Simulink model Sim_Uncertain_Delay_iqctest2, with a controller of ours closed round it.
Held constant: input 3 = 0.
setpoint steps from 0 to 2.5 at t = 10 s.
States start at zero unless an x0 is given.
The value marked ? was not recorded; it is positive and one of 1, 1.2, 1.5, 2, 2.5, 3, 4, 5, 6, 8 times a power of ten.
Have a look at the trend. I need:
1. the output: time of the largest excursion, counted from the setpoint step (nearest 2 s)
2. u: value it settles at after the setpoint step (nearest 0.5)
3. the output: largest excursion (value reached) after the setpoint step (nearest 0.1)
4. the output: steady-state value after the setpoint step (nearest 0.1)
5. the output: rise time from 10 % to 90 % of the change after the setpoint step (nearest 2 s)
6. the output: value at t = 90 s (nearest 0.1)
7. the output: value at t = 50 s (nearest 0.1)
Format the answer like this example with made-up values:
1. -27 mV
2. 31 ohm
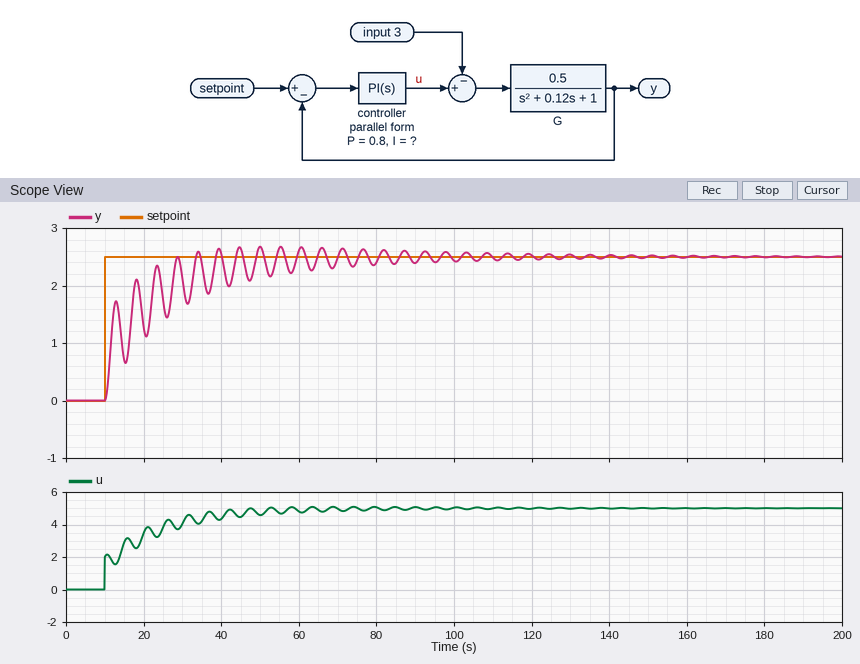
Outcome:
1. 40 s
2. 5.0
3. 2.7
4. 2.5
5. 12 s
6. 2.4
7. 2.7
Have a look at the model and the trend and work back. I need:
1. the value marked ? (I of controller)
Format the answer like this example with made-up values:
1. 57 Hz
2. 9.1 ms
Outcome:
1. 0.2
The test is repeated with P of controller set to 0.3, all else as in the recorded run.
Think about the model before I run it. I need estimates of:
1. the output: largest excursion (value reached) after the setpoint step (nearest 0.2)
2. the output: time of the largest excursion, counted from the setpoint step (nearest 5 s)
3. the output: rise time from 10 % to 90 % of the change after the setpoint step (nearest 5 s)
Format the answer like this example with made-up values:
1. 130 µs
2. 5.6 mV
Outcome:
1. 2.6
2. 50 s
3. 20 s
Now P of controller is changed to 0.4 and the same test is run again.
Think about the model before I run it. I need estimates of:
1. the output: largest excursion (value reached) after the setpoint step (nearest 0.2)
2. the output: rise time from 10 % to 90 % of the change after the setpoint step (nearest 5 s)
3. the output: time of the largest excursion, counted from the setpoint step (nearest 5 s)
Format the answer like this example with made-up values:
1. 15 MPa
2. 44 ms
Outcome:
1. 2.6
2. 20 s
3. 50 s
